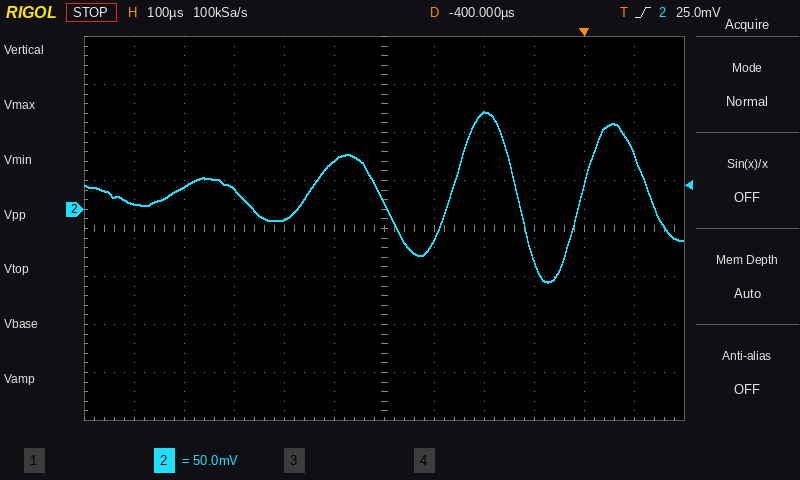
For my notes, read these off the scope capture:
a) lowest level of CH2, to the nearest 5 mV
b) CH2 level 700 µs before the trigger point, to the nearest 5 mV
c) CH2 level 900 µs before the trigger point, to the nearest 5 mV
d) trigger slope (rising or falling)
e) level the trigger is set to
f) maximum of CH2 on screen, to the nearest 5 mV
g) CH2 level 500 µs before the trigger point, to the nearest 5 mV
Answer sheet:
-75 mV
20 mV
5 mV
rising
25.0 mV
100 mV
50 mV
